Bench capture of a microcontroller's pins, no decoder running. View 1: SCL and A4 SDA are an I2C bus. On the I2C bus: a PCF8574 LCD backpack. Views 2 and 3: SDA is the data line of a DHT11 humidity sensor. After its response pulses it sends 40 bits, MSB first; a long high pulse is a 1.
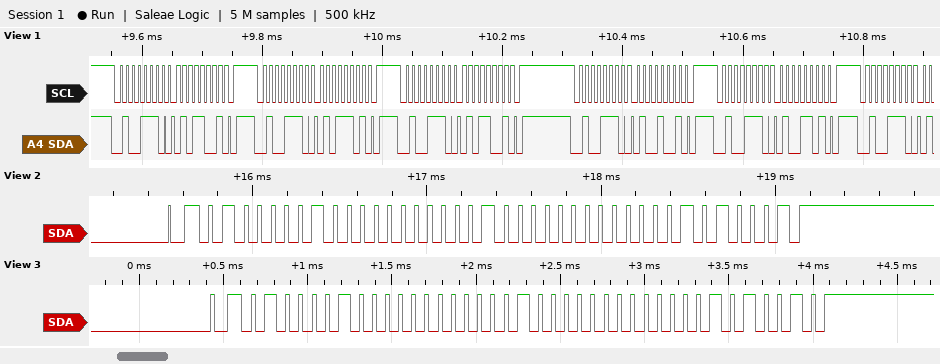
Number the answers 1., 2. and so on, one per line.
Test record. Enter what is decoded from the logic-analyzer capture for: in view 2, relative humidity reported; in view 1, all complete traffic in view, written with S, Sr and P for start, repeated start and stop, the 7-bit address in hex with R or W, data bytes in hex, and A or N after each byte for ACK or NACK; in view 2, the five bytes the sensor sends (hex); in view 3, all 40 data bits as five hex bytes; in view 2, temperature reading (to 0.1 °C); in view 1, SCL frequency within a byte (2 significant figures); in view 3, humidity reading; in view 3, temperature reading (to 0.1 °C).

1. 65 %
2. S 27W A 59 A P S 27W A 5D A P S 27W A 59 A P S 27W A 49 A P S 27W A 4D A P S 27W A
3. 41 00 10 00 51
4. 42 00 10 00 52
5. 16.0 °C
6. 100 kHz
7. 66 %
8. 16.0 °C
